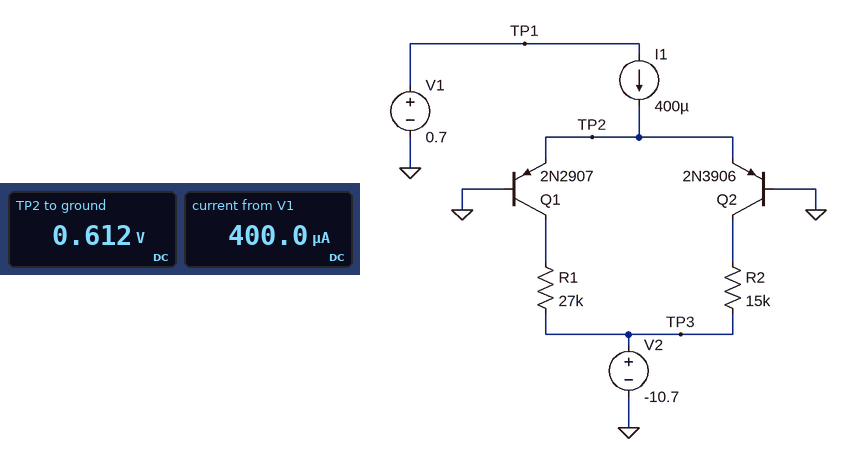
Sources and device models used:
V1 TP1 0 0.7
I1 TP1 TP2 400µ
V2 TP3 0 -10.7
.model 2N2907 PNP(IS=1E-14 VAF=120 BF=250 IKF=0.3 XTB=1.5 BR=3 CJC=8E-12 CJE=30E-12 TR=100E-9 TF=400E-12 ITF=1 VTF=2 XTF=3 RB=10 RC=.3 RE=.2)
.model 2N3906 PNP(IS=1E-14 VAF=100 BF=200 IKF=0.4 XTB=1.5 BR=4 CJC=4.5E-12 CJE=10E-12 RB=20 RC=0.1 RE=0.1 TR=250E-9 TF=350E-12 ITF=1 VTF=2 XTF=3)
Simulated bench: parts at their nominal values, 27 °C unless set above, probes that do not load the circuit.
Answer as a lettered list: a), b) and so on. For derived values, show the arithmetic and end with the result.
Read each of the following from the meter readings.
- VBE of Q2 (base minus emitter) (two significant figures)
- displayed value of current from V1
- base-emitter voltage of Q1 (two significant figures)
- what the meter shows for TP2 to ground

a) 0 V - 612 mV = -610 mV
b) 400.0 µA
c) 0 V - 612 mV = -610 mV
d) 0.612 V
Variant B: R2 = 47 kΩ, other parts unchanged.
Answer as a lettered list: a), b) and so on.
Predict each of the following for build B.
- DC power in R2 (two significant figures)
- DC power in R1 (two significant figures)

a) 1.8 mW
b) 1.1 mW
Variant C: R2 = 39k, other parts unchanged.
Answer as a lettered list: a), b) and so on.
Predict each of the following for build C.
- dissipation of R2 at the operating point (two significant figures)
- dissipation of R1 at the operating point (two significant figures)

a) 1.5 mW
b) 1.1 mW
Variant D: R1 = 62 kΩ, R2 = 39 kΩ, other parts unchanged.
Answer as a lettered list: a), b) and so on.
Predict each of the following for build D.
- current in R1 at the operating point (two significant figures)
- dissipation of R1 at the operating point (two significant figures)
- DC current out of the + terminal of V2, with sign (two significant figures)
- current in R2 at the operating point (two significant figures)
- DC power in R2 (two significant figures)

a) 180 µA
b) 2.0 mW
c) -390 µA
d) 210 µA
e) 1.7 mW
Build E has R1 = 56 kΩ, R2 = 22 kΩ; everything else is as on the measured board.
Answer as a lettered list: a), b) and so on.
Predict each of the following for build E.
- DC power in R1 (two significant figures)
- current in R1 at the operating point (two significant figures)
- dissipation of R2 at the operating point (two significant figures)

a) 2.1 mW
b) 190 µA
c) 930 µW
